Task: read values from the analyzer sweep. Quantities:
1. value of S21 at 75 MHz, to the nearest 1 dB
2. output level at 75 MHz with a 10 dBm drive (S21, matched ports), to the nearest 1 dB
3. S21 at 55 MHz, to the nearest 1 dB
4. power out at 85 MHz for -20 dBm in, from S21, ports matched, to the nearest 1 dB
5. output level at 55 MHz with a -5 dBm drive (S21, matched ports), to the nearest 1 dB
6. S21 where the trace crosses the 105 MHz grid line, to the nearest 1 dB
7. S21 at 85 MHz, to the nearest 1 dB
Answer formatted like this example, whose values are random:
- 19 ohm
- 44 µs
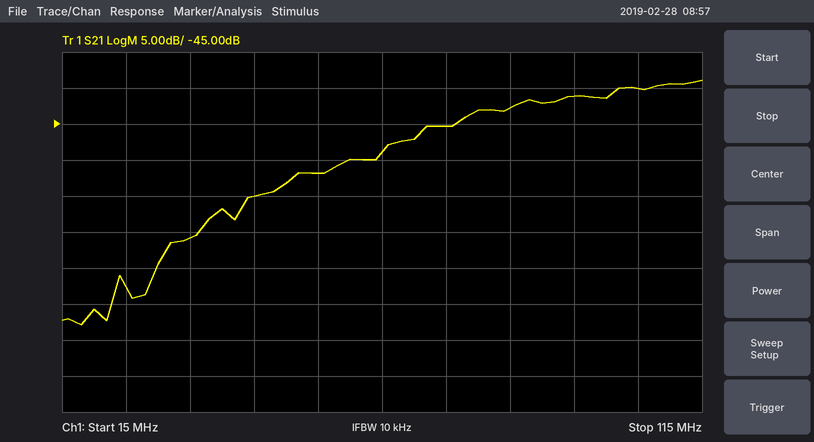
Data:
- -45 dB
- -35 dBm
- -52 dB
- -63 dBm
- -57 dBm
- -40 dB
- -43 dB
